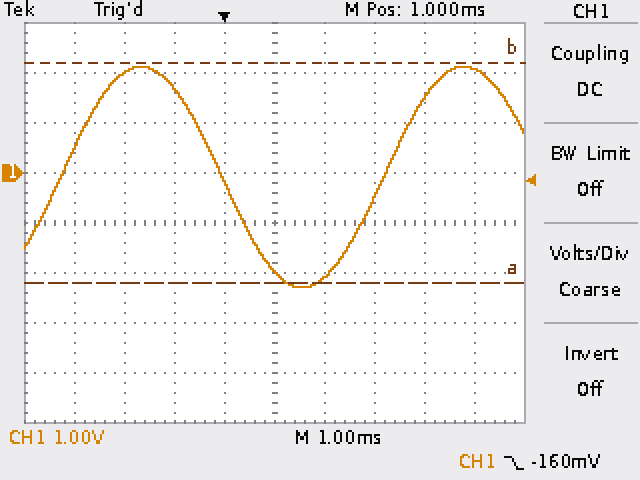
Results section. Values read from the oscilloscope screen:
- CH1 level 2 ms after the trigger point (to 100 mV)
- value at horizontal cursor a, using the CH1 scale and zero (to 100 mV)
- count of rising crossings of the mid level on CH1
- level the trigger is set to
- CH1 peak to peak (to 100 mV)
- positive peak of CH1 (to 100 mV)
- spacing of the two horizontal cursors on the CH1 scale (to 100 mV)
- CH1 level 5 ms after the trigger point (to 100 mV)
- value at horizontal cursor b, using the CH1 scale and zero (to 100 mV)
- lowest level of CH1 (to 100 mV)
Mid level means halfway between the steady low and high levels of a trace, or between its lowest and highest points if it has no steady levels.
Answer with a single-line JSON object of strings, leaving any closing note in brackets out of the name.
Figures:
{"CH1 level 2 ms after the trigger point": "-2.1 V", "value at horizontal cursor a, using the CH1 scale and zero": "-2.2 V", "count of rising crossings of the mid level on CH1": "2", "level the trigger is set to": "-160 mV", "CH1 peak to peak": "4.4 V", "positive peak of CH1": "2.1 V", "spacing of the two horizontal cursors on the CH1 scale": "4.4 V", "CH1 level 5 ms after the trigger point": "2.1 V", "value at horizontal cursor b, using the CH1 scale and zero": "2.2 V", "lowest level of CH1": "-2.3 V"}
